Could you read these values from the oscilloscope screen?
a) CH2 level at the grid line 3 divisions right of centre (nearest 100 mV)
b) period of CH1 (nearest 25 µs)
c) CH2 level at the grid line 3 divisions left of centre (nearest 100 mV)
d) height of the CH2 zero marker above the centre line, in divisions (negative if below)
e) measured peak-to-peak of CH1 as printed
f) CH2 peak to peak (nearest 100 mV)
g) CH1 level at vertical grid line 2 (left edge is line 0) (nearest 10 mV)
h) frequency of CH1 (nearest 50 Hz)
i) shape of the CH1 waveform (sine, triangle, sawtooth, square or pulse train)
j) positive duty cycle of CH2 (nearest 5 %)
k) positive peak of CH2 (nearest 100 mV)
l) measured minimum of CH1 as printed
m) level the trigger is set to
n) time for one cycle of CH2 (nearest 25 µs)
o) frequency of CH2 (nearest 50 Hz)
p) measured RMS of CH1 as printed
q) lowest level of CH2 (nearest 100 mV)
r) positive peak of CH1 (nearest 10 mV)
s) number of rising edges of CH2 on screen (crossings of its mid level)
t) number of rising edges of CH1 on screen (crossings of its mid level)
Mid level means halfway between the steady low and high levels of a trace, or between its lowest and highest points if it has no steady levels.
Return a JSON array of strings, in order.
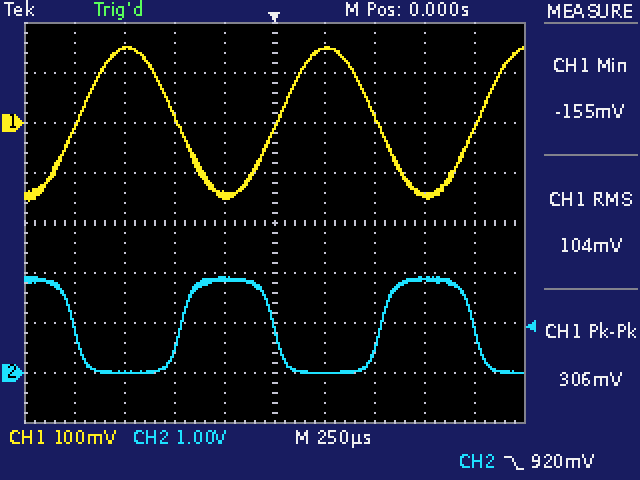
["1.9 V", "1.000 ms", "0.0 V", "-3.0 div", "306 mV", "1.9 V", "150 mV", "1.00 kHz", "sine", "45 %", "1.9 V", "-155 mV", "920 mV", "1.000 ms", "1.00 kHz", "104 mV", "0.0 V", "150 mV", "2", "3"]
